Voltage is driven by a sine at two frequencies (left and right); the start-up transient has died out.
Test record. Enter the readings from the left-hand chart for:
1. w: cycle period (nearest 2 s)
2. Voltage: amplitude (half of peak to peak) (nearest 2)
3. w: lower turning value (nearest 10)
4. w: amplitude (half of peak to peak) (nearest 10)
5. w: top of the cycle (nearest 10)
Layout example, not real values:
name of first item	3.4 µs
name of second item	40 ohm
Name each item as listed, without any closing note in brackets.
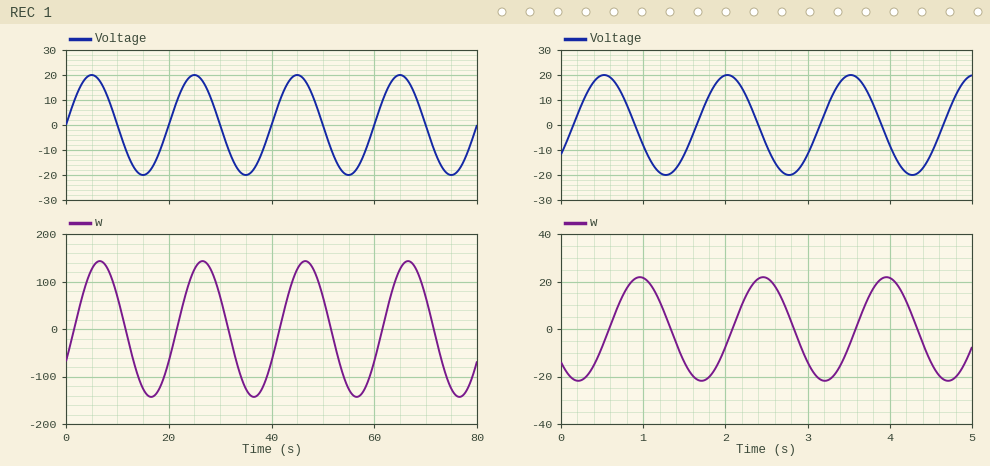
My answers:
w: cycle period	20 s
Voltage: amplitude (half of peak to peak)	20
w: lower turning value	-140
w: amplitude (half of peak to peak)	140
w: top of the cycle	140
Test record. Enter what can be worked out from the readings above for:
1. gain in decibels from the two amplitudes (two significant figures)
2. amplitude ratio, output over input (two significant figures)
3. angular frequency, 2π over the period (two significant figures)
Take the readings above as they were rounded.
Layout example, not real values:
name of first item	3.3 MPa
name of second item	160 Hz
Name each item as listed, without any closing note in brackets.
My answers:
gain in decibels from the two amplitudes	17 dB
amplitude ratio, output over input	7.0
angular frequency, 2π over the period	0.31 rad/s
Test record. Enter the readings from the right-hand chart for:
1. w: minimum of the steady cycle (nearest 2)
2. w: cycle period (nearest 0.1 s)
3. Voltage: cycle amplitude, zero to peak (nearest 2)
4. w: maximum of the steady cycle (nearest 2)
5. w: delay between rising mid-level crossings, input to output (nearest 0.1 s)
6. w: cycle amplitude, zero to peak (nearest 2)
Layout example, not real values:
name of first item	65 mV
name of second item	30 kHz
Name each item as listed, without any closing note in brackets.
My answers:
w: minimum of the steady cycle	-22
w: cycle period	1.5 s
Voltage: cycle amplitude, zero to peak	20
w: maximum of the steady cycle	22
w: delay between rising mid-level crossings, input to output	0.4 s
w: cycle amplitude, zero to peak	22
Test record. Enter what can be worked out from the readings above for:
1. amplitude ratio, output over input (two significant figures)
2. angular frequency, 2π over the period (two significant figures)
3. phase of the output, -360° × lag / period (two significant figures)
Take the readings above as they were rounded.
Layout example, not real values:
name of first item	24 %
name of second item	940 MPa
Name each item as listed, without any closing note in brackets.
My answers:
amplitude ratio, output over input	1.1
angular frequency, 2π over the period	4.2 rad/s
phase of the output, -360° × lag / period	-96°
